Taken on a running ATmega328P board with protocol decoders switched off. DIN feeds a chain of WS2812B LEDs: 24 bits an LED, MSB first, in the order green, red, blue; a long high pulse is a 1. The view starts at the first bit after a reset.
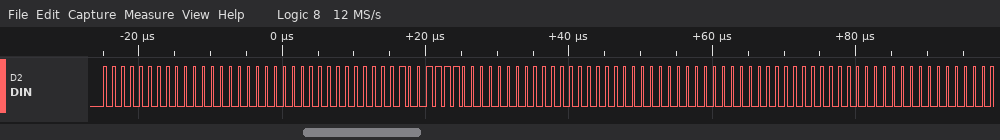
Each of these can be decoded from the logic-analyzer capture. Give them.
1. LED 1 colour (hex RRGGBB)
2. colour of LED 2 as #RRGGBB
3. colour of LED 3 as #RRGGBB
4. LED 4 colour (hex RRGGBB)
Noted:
#000000
#4F0000
#000000
#000000
